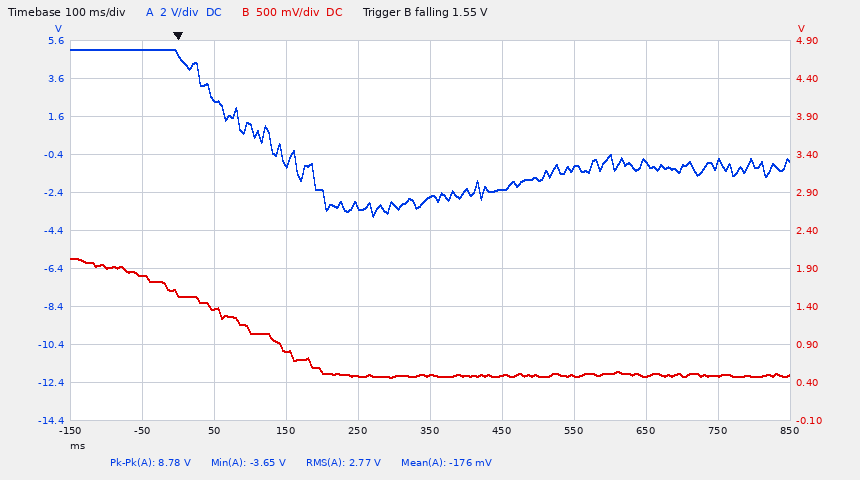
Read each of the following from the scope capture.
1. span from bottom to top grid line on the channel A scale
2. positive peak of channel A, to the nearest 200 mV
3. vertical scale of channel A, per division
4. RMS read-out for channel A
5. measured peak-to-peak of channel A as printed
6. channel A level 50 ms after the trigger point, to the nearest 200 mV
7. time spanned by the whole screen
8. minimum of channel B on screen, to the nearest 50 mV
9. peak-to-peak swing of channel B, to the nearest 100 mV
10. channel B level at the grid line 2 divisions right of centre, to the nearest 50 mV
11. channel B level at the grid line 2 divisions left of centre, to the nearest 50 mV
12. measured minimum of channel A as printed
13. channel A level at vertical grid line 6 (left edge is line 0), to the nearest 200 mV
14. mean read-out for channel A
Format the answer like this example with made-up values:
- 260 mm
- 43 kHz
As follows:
- 20 V
- 5.2 V
- 2 V
- 2.77 V
- 8.78 V
- 2.6 V
- 1 s
- 450 mV
- 1.60 V
- 500 mV
- 800 mV
- -3.65 V
- -2.2 V
- -176 mV
